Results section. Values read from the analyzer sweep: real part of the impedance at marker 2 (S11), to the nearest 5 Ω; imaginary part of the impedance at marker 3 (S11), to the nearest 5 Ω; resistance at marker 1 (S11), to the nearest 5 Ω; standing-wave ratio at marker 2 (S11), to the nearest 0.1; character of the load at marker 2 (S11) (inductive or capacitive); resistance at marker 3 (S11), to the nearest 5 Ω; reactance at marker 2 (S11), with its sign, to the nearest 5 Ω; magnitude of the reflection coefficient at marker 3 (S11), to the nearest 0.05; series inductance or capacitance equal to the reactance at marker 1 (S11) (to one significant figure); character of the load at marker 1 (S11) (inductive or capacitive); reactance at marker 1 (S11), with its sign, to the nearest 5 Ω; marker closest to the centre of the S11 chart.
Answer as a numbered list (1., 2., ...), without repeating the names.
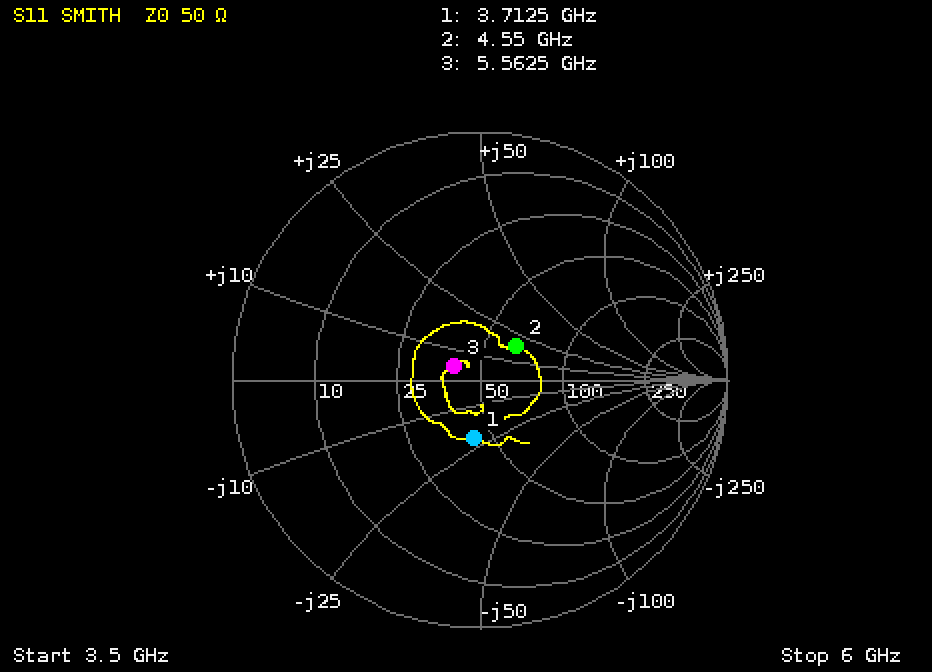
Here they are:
1. 65 Ω
2. +5 Ω
3. 45 Ω
4. 1.5
5. inductive
6. 40 Ω
7. +20 Ω
8. 0.10
9. 2 pF
10. capacitive
11. -20 Ω
12. marker 3
